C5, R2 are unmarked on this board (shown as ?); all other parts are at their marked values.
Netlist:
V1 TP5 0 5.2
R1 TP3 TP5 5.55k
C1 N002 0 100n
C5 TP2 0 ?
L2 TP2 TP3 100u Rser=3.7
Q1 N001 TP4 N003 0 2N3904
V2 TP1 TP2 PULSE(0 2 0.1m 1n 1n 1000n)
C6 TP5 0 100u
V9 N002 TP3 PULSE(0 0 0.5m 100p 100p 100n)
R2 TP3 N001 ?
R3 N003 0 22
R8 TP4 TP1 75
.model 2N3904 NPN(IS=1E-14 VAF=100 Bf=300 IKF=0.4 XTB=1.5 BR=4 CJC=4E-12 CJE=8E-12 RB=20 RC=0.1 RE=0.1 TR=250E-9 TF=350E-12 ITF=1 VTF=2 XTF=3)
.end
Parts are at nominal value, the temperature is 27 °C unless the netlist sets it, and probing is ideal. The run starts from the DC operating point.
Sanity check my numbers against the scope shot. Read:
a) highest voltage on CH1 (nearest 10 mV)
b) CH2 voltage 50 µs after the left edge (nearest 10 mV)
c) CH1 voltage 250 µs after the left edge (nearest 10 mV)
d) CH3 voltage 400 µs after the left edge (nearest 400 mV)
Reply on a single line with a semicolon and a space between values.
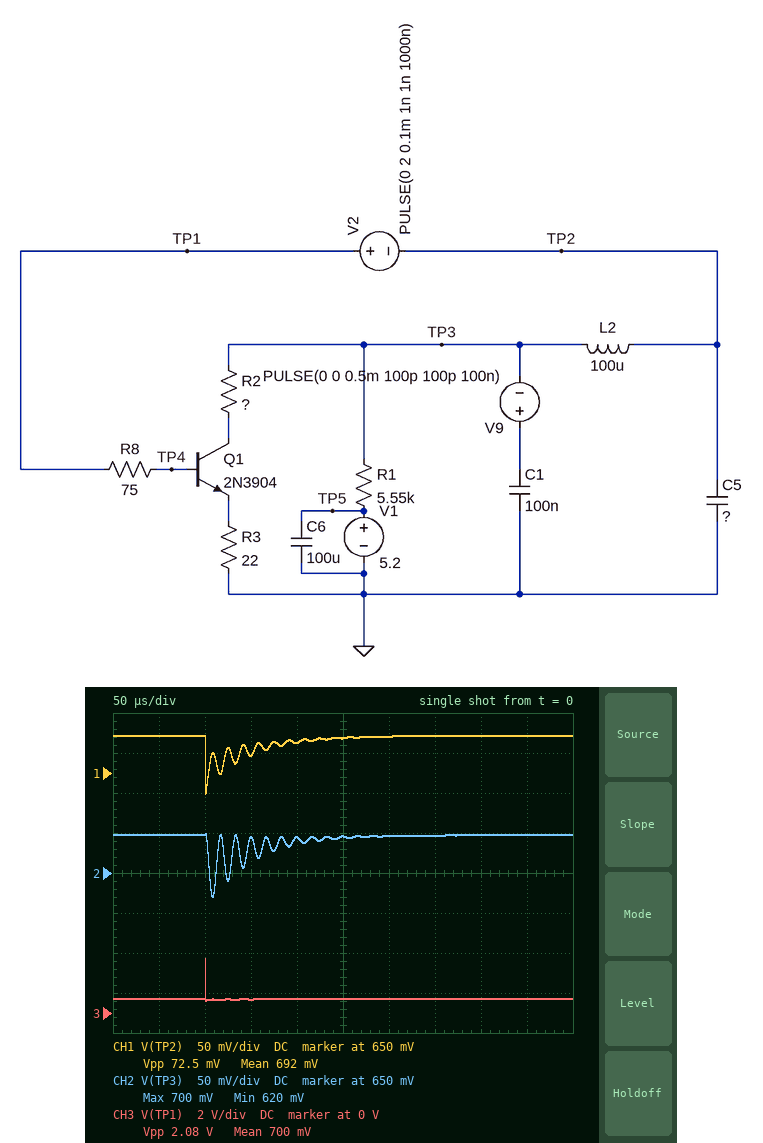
700 mV; 700 mV; 690 mV; 800 mV
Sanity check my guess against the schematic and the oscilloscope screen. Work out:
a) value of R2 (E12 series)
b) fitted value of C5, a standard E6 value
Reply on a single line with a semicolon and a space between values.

1 kΩ; 220 nF
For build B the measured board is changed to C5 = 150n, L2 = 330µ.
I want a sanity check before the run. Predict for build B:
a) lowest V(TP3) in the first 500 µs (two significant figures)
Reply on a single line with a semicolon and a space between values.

610 mV
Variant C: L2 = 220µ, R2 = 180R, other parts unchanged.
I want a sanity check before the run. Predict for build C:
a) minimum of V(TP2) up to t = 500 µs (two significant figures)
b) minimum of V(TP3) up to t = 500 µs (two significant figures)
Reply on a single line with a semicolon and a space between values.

490 mV; 310 mV
